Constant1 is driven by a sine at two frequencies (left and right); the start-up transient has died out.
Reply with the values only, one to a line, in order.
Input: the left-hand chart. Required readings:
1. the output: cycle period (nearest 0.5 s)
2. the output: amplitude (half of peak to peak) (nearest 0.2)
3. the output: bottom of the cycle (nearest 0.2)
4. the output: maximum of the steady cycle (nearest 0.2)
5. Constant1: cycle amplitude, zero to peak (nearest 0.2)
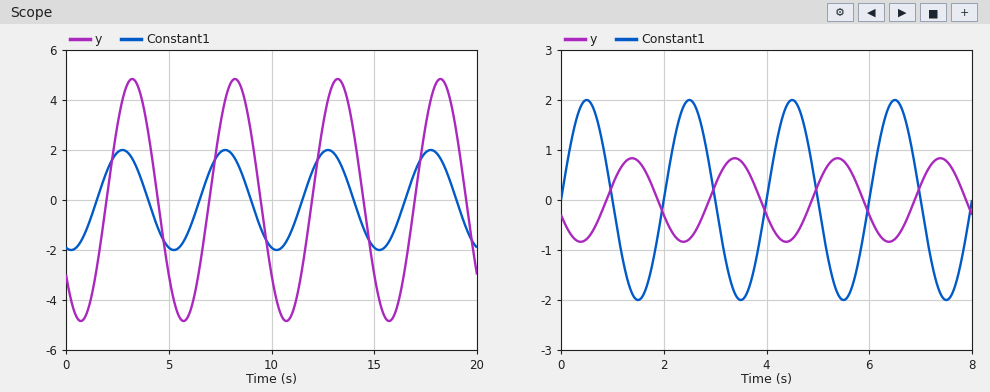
5.0 s
4.8
-4.8
4.8
2.0
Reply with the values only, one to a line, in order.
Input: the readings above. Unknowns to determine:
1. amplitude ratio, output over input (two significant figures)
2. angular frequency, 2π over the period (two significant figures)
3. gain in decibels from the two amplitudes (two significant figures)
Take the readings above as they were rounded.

2.4
1.3 rad/s
7.6 dB
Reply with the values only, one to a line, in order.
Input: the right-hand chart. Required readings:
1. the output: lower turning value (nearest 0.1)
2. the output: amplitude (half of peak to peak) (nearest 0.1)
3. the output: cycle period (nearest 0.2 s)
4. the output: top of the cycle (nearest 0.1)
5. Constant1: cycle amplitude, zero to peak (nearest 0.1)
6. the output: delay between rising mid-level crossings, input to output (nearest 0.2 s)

-0.8
0.8
2.0 s
0.8
2.0
0.8 s
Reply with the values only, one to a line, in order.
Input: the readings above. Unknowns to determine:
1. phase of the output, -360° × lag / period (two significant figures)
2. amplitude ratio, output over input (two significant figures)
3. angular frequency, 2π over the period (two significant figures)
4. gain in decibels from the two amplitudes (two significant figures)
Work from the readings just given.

-140°
0.40
3.1 rad/s
-8.0 dB
